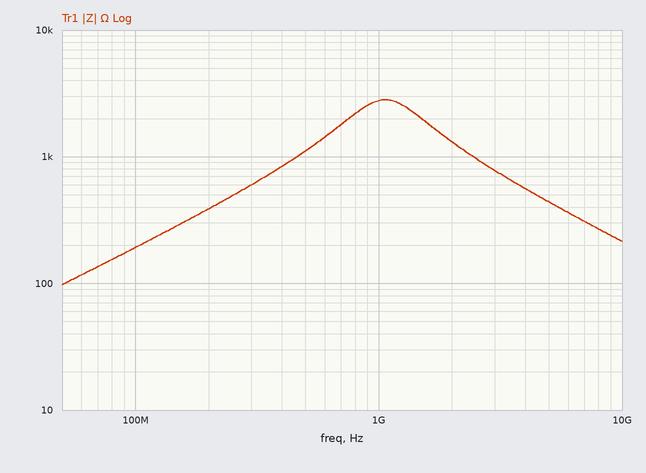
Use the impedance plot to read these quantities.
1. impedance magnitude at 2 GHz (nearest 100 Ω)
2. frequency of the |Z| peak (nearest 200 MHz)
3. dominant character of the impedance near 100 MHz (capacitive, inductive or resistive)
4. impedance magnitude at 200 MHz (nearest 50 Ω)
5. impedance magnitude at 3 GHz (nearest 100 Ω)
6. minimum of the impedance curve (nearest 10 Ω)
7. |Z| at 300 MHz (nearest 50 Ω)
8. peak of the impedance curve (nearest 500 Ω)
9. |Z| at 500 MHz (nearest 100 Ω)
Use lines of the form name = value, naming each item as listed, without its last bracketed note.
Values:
impedance magnitude at 2 GHz = 1.3 kΩ
frequency of the |Z| peak = 1.0 GHz
dominant character of the impedance near 100 MHz = inductive
impedance magnitude at 200 MHz = 400 Ω
impedance magnitude at 3 GHz = 800 Ω
minimum of the impedance curve = 100 Ω
|Z| at 300 MHz = 600 Ω
peak of the impedance curve = 3.0 kΩ
|Z| at 500 MHz = 1.1 kΩ
